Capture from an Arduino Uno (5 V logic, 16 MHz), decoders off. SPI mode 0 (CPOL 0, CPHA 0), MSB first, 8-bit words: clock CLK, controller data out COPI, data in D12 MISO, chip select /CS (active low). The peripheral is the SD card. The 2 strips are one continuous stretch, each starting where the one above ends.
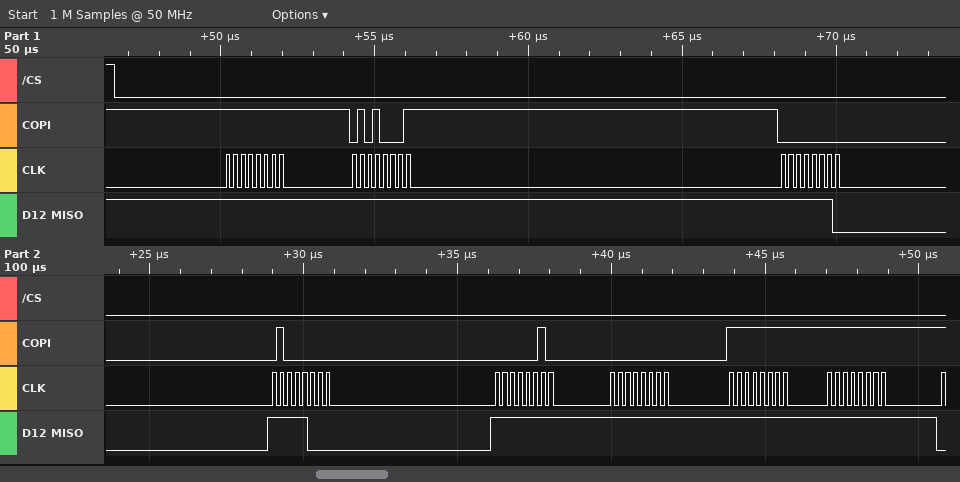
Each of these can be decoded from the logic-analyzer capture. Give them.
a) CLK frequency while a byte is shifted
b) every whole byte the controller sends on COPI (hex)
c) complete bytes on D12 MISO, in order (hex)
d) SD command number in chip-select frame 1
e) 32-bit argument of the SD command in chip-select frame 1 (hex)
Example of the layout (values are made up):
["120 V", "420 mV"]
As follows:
["4 MHz", "FF 51 00 40 02 00 FF FF", "FF FF FE F8 FF FF FF FF", "CMD17", "0x00400200"]
